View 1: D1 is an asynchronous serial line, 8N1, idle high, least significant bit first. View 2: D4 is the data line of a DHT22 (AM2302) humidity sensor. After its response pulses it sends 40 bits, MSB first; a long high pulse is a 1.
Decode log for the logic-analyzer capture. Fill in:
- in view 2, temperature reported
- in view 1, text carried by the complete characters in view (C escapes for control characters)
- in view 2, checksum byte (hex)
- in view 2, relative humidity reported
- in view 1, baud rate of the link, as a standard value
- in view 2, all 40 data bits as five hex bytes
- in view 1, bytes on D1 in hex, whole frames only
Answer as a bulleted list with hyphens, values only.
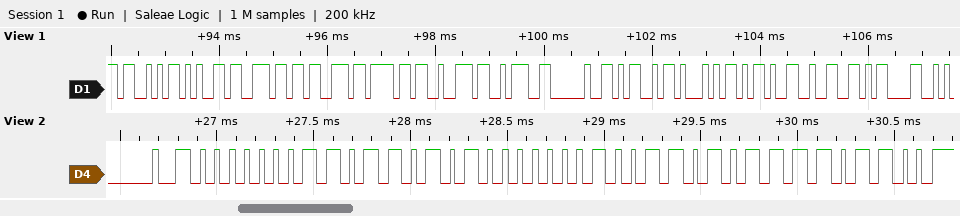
- 30.9 °C
- "Sensor: MQ-2\r"
- 0xEC
- 43.7 %
- 9600 baud
- 01 B5 01 35 EC
- 53 65 6E 73 6F 72 3A 20 4D 51 2D 32 0D
